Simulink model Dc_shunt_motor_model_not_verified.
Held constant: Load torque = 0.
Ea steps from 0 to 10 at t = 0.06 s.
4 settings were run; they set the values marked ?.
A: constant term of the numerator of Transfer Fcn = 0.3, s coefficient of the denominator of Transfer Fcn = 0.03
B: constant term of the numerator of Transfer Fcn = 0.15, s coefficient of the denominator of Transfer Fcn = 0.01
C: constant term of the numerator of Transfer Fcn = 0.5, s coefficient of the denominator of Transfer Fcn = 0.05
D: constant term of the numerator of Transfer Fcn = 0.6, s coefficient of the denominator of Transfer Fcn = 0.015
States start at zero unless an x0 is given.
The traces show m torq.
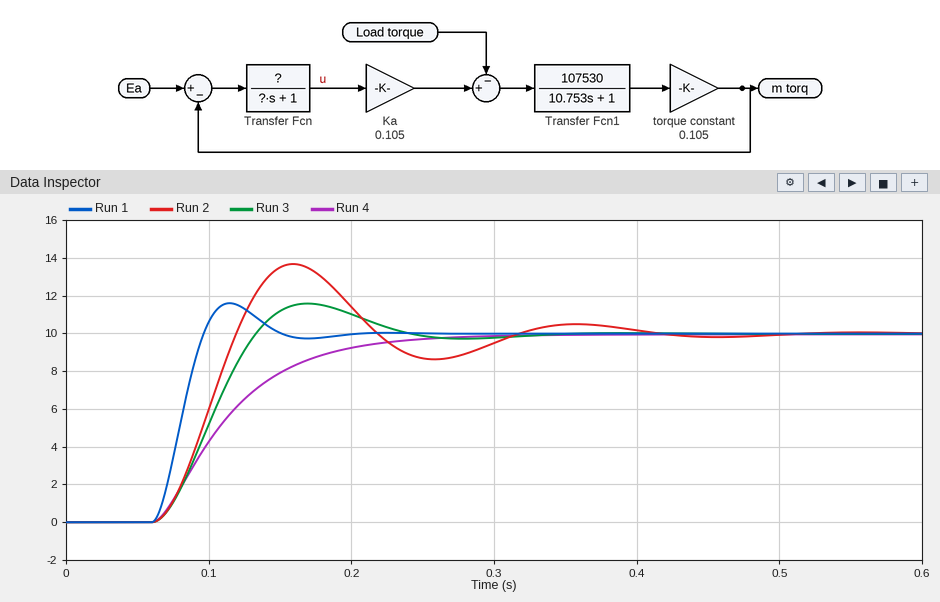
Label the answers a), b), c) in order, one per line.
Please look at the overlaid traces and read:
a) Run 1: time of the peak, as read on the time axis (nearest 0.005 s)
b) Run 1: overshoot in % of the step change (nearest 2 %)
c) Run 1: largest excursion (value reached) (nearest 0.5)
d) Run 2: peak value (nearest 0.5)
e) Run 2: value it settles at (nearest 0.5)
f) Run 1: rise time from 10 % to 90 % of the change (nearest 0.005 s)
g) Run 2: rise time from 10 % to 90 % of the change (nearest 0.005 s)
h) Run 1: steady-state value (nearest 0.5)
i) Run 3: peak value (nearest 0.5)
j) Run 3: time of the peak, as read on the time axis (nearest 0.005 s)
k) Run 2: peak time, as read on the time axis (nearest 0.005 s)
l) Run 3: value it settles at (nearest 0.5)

a) 0.115 s
b) 16 %
c) 11.5
d) 13.5
e) 10.0
f) 0.025 s
g) 0.040 s
h) 10.0
i) 11.5
j) 0.170 s
k) 0.160 s
l) 10.0
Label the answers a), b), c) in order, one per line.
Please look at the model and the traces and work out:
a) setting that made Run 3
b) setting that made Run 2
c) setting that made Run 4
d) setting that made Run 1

a) A
b) C
c) B
d) D
